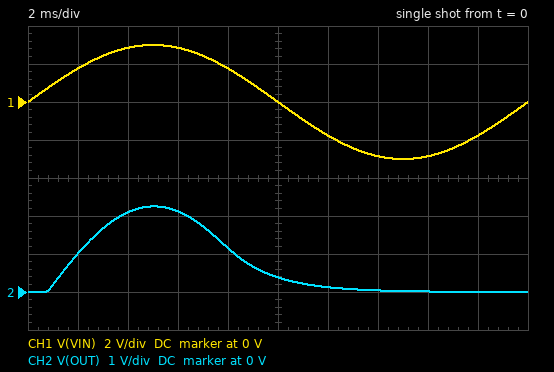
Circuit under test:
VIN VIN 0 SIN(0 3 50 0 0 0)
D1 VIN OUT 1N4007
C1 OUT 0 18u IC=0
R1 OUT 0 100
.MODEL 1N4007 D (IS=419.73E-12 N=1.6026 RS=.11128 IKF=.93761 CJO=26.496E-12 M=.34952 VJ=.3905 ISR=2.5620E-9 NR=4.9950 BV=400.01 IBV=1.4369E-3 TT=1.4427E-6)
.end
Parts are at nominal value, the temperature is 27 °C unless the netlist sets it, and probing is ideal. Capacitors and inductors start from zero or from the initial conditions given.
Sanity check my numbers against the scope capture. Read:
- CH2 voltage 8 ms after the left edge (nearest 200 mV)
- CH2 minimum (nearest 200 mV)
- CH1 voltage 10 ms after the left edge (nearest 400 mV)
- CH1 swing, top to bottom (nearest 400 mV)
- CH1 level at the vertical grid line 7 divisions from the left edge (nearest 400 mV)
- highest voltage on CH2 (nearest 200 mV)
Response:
1.2 V
0 V
0 V
6.0 V
-2.8 V
2.2 V
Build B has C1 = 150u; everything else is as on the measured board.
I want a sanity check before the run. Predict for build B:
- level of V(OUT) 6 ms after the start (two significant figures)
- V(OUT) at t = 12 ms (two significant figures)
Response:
2.2 V
1.5 V
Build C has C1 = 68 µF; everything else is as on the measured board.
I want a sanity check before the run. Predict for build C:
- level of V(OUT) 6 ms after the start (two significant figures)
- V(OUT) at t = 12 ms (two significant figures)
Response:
2.2 V
910 mV
